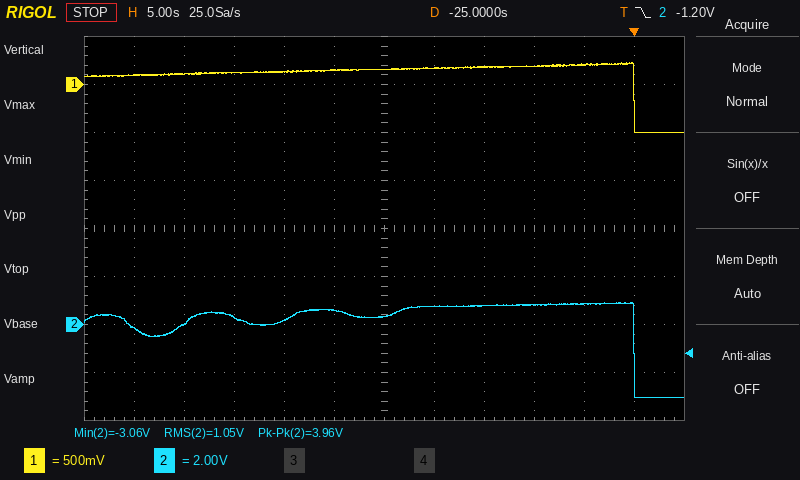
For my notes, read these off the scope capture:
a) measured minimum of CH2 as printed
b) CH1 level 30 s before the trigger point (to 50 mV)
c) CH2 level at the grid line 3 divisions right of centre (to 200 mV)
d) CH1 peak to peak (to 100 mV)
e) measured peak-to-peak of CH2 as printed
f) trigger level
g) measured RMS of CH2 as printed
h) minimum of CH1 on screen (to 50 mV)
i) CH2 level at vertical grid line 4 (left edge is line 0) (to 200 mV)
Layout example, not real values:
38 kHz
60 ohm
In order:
-3.06 V
150 mV
800 mV
700 mV
3.96 V
-1.20 V
1.05 V
-500 mV
200 mV
